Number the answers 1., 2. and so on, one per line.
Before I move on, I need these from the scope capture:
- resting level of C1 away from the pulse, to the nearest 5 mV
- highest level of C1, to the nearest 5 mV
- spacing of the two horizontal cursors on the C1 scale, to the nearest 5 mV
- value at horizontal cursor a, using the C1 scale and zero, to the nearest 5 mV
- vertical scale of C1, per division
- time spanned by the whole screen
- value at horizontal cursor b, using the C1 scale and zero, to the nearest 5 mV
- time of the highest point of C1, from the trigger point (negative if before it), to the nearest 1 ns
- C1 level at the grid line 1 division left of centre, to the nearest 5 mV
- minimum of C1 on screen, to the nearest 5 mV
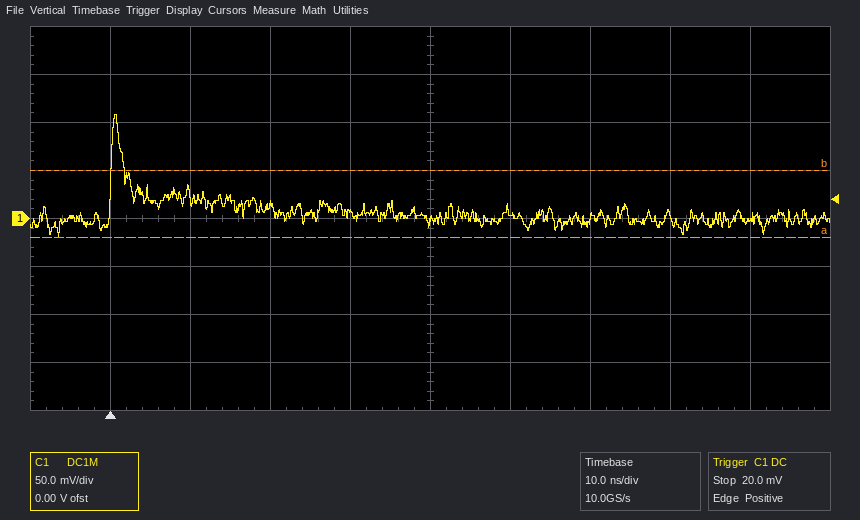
1. 0 mV
2. 110 mV
3. 70 mV
4. -20 mV
5. 50 mV
6. 100 ns
7. 50 mV
8. +1 ns
9. 5 mV
10. -20 mV
